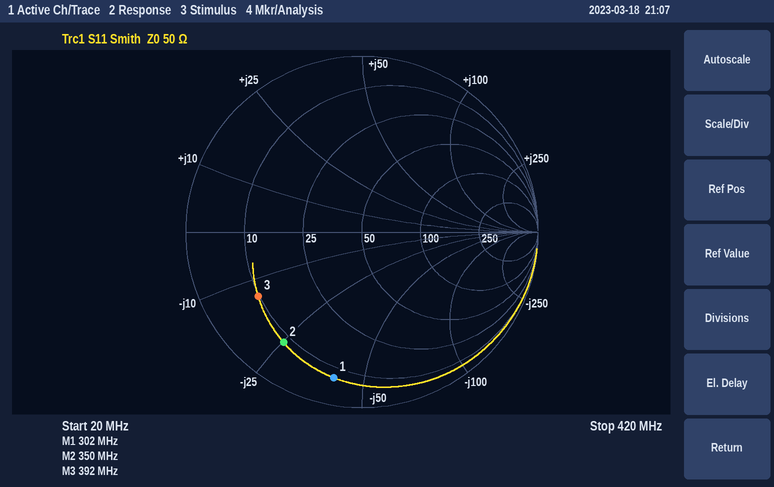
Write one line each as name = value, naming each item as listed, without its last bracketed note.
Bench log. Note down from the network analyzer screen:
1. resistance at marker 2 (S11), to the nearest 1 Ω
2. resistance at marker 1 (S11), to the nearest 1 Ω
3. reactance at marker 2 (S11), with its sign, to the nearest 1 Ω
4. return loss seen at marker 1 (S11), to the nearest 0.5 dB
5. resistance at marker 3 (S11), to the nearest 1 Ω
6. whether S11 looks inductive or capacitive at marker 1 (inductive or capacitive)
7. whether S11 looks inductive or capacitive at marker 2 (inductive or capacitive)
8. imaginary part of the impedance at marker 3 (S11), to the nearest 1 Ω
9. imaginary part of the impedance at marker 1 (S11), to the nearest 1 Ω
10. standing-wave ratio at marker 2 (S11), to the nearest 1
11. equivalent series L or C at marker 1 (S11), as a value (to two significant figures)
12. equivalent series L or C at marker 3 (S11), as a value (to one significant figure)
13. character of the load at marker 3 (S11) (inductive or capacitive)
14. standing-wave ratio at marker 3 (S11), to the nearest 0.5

resistance at marker 2 (S11), to the nearest 1 Ω = 8 Ω
resistance at marker 1 (S11), to the nearest 1 Ω = 7 Ω
reactance at marker 2 (S11), with its sign, to the nearest 1 Ω = -25 Ω
return loss seen at marker 1 (S11), to the nearest 0.5 dB = 1.5 dB
resistance at marker 3 (S11), to the nearest 1 Ω = 10 Ω
whether S11 looks inductive or capacitive at marker 1 = capacitive
whether S11 looks inductive or capacitive at marker 2 = capacitive
imaginary part of the impedance at marker 3 (S11), to the nearest 1 Ω = -14 Ω
imaginary part of the impedance at marker 1 (S11), to the nearest 1 Ω = -41 Ω
standing-wave ratio at marker 2 (S11), to the nearest 1 = 8
equivalent series L or C at marker 1 (S11), as a value = 13 pF
equivalent series L or C at marker 3 (S11), as a value = 30 pF
character of the load at marker 3 (S11) = capacitive
standing-wave ratio at marker 3 (S11), to the nearest 0.5 = 5.5
